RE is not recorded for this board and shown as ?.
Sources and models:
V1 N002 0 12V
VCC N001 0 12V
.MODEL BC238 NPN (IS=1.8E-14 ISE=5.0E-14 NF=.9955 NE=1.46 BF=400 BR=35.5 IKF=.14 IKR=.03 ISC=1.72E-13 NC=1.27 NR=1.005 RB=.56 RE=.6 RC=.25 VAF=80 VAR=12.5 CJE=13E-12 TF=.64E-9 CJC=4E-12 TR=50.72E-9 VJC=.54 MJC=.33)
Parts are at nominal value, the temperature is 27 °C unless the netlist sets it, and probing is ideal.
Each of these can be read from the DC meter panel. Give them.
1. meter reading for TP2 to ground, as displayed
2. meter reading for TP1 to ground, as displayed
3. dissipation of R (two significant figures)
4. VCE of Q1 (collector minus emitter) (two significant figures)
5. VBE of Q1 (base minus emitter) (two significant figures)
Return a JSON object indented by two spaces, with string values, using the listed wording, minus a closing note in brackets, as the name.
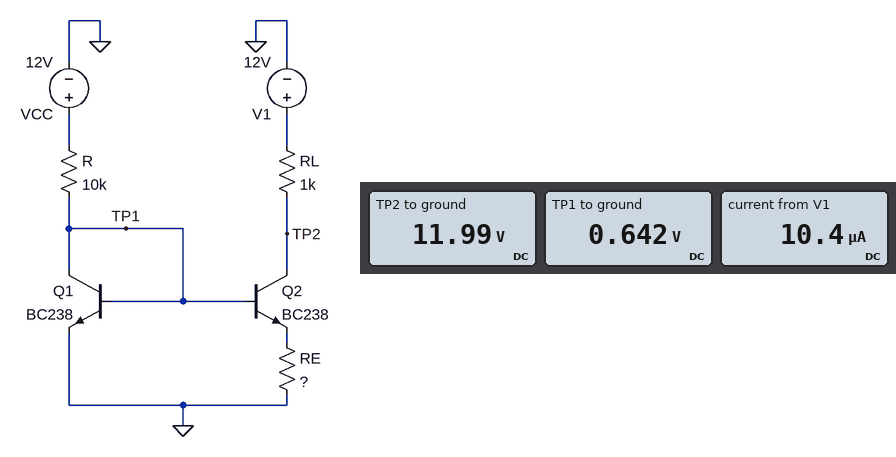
{
  "meter reading for TP2 to ground, as displayed": "11.99 V",
  "meter reading for TP1 to ground, as displayed": "0.642 V",
  "dissipation of R": "13 mW",
  "VCE of Q1 (collector minus emitter)": "640 mV",
  "VBE of Q1 (base minus emitter)": "640 mV"
}
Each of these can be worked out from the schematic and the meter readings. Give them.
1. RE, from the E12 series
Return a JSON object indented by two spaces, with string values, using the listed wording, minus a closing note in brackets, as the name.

{
  "RE, from the E12 series": "12 kΩ"
}
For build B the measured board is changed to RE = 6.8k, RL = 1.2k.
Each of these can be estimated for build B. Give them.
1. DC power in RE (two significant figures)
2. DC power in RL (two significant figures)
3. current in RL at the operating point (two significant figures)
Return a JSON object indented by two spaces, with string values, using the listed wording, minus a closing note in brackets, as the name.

{
  "DC power in RE": "1.9 µW",
  "DC power in RL": "330 nW",
  "current in RL at the operating point": "17 µA"
}
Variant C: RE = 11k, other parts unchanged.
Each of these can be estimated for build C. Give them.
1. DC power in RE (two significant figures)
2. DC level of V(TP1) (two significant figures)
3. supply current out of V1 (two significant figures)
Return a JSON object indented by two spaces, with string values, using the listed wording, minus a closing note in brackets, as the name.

{
  "DC power in RE": "1.4 µW",
  "DC level of V(TP1)": "640 mV",
  "supply current out of V1": "11 µA"
}
